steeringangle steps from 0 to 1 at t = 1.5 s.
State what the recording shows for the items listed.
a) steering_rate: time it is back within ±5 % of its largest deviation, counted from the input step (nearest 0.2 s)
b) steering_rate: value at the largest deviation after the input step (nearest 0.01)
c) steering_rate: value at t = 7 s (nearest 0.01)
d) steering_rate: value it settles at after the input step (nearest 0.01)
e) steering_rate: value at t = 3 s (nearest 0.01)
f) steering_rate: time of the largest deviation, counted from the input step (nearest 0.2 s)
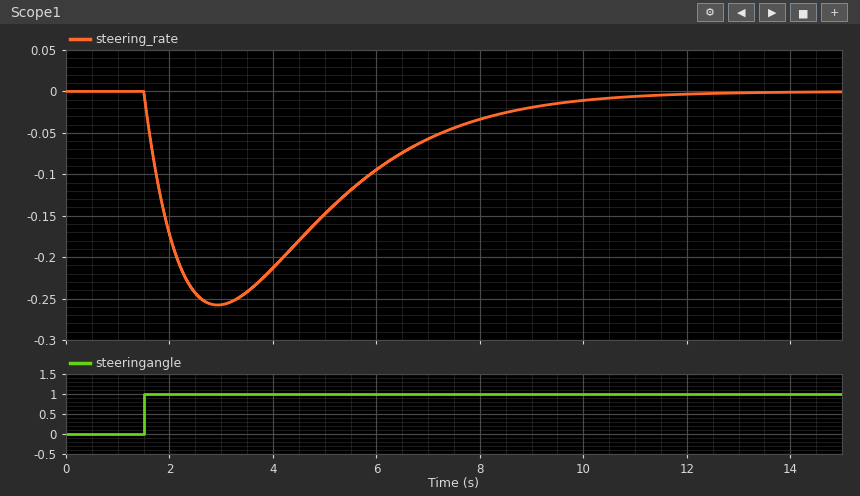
8.2 s
-0.26
-0.06
0.00
-0.26
1.4 s
